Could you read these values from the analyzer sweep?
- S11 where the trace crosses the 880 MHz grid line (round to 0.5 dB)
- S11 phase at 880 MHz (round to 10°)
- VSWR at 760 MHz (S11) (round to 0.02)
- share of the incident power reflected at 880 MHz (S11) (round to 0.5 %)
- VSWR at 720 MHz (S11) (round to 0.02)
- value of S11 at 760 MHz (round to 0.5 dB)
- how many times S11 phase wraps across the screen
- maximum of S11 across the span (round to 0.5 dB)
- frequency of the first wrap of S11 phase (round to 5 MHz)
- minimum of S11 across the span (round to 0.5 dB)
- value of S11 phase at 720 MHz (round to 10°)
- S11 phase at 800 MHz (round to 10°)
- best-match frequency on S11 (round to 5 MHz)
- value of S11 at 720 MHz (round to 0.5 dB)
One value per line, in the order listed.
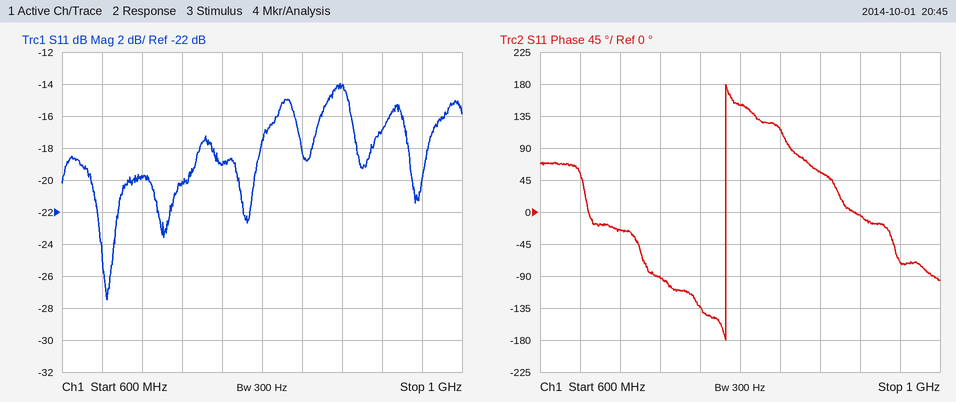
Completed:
-14.0 dB
60°
1.26
4.0 %
1.22
-19.0 dB
1
-14.0 dB
785 MHz
-27.5 dB
-90°
150°
645 MHz
-20.0 dB
